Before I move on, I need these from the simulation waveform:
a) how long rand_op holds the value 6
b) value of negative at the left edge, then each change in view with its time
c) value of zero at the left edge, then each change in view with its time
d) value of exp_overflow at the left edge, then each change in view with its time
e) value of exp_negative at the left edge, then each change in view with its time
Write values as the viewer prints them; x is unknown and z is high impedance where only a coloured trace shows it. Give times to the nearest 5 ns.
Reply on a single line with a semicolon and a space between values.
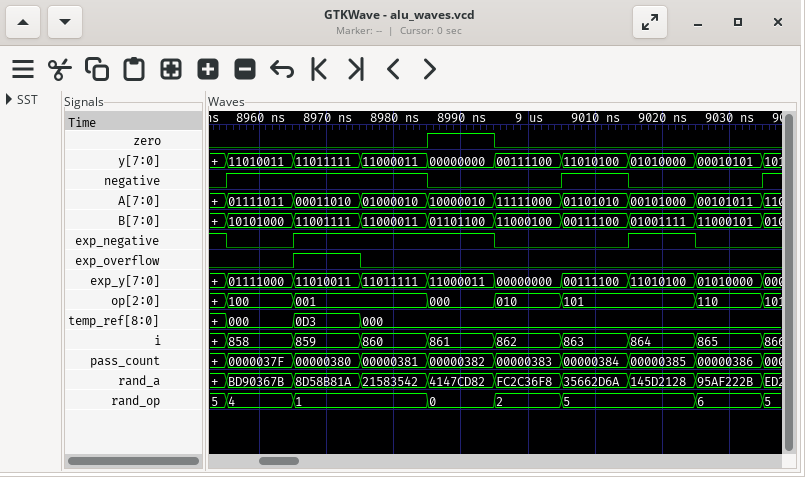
10 ns; 0, 1 at 8955 ns, 0 at 8985 ns, 1 at 9005 ns, 0 at 9015 ns, 1 at 9035 ns; 0, 1 at 8985 ns, 0 at 8995 ns; 0, 1 at 8965 ns, 0 at 8975 ns; 1, 0 at 8955 ns, 1 at 8965 ns, 0 at 8995 ns, 1 at 9015 ns, 0 at 9025 ns
